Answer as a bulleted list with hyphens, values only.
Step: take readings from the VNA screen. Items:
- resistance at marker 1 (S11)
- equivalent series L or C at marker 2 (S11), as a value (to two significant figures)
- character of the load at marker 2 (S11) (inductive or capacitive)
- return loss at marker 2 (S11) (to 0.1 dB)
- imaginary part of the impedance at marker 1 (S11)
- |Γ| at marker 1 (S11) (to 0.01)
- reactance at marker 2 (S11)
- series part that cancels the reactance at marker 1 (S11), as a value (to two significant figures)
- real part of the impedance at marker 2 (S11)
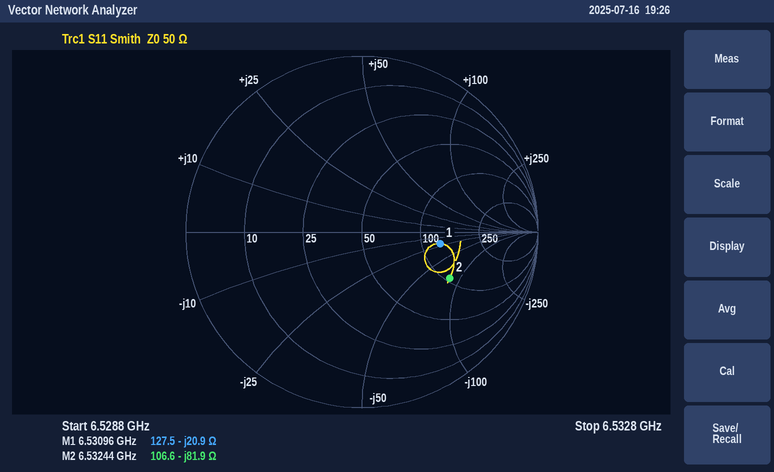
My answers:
- 127.5 Ω
- 300 fF
- capacitive
- 5.0 dB
- -20.9 Ω
- 0.45
- -81.9 Ω
- 510 pH
- 106.6 Ω
